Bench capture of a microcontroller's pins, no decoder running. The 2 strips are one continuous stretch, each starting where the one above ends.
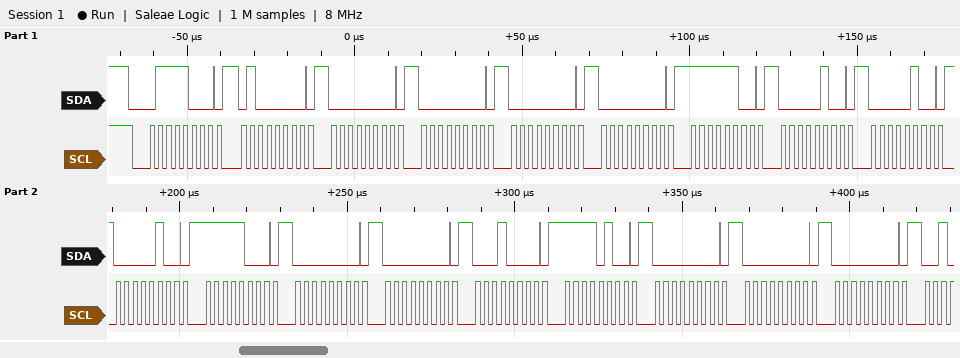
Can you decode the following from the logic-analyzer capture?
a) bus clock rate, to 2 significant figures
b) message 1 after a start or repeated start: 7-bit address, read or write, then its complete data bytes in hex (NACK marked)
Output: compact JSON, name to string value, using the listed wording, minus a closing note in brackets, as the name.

{"bus clock rate, to 2 significant figures": "400 kHz", "message 1 after a start or repeated start: 7-bit address, read or write, then its complete data bytes in hex": "0x3C write: 40 00 00 00 00 FC 04 04 04 F8 00 00 10 F4 00 00 00"}
